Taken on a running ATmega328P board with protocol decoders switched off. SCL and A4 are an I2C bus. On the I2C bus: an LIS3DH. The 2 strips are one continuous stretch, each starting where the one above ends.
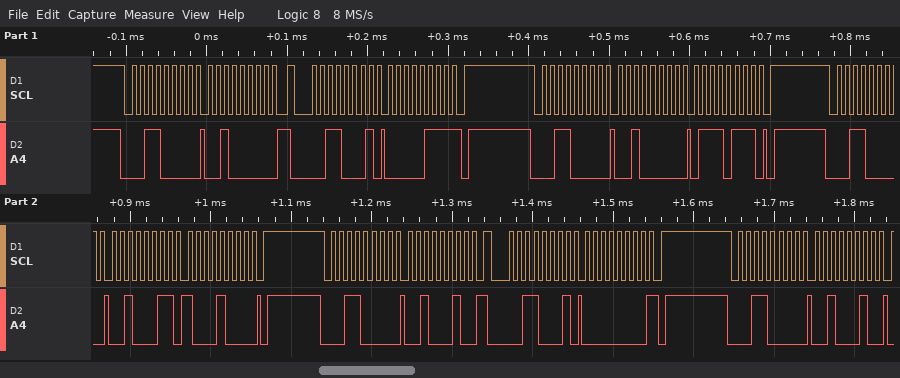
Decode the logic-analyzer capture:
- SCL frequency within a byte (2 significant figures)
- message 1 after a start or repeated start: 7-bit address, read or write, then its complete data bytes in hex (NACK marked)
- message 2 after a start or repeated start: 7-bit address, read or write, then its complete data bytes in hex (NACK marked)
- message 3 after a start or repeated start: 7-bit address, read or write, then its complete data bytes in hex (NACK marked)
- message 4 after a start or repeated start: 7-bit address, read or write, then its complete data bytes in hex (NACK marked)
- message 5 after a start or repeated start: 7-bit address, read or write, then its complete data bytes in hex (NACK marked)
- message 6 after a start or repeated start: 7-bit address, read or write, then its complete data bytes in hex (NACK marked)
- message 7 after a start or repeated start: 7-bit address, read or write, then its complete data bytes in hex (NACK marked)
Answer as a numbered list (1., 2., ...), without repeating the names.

1. 100 kHz
2. 0x18 write: 20
3. 0x18 read: 07 NACK
4. 0x18 write: 20 77
5. 0x18 write: 23 88
6. 0x18 write: 22
7. 0x18 read: 00 NACK
8. 0x18 write: 22
